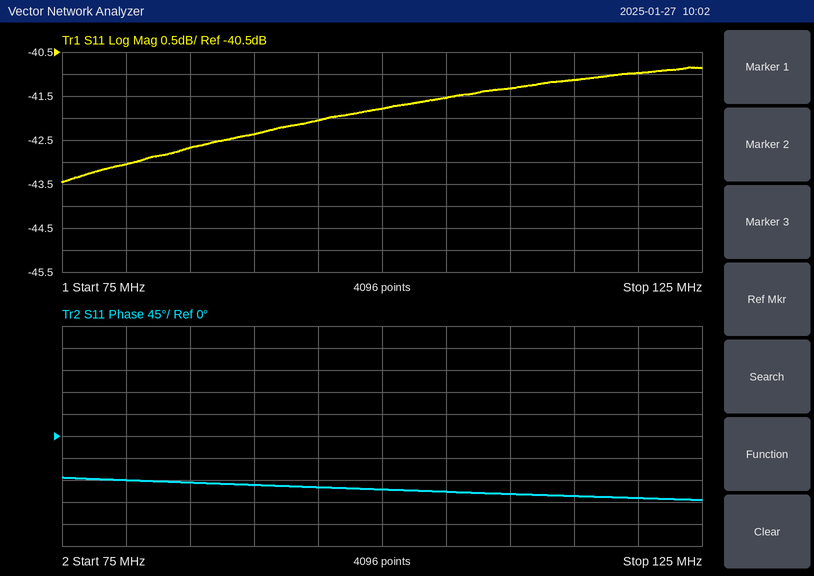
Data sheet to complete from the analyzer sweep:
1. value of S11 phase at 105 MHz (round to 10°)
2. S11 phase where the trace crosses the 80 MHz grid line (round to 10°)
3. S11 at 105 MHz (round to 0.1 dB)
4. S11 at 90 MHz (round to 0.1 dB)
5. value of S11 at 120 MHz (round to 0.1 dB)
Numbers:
-110°
-90°
-41.5 dB
-42.4 dB
-41.0 dB
